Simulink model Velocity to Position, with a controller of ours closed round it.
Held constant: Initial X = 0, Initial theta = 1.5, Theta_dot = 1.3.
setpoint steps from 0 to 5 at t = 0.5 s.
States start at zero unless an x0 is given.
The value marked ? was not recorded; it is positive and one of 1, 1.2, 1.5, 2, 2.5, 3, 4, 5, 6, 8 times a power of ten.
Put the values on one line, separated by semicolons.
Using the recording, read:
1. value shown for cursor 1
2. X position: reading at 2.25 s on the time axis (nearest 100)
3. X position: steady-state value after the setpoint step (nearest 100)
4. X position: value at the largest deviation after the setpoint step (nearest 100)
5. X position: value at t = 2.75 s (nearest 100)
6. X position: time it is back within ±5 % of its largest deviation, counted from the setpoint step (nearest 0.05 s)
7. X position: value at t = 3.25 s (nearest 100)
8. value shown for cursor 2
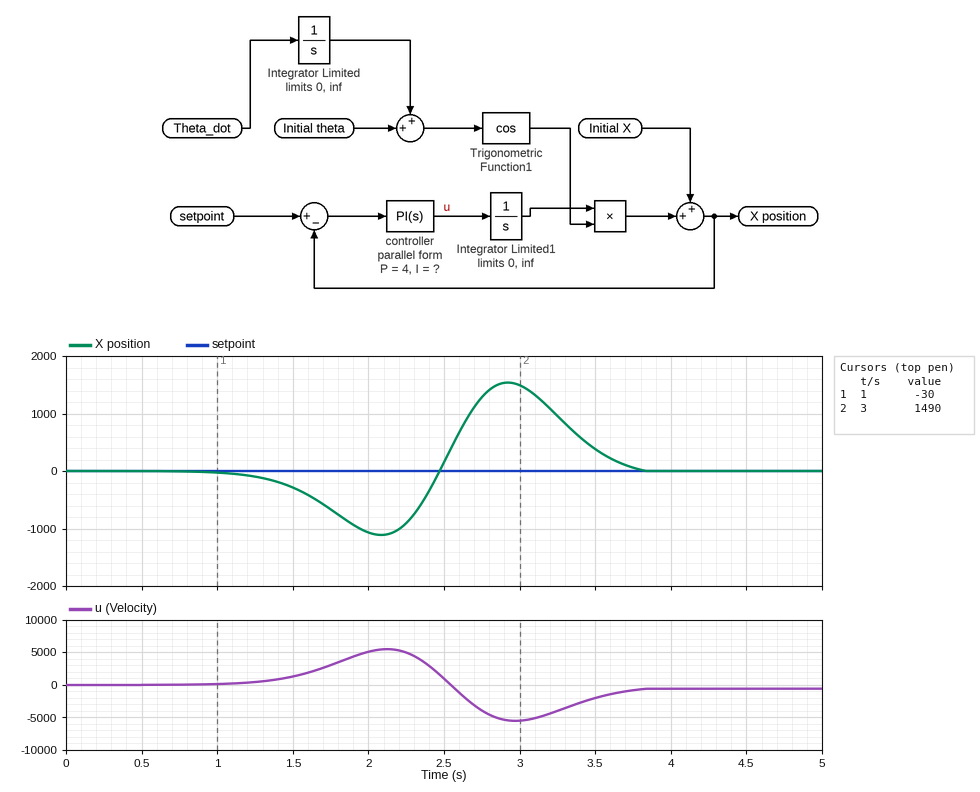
-30; -900; 0; 1500; 1300; 3.25 s; 1000; 1490
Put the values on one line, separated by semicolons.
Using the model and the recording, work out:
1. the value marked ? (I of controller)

2
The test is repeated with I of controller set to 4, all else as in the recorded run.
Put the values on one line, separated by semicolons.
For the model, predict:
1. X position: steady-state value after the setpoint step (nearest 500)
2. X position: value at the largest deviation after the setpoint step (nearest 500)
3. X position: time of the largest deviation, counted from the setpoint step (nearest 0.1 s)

0; 3000; 2.4 s
